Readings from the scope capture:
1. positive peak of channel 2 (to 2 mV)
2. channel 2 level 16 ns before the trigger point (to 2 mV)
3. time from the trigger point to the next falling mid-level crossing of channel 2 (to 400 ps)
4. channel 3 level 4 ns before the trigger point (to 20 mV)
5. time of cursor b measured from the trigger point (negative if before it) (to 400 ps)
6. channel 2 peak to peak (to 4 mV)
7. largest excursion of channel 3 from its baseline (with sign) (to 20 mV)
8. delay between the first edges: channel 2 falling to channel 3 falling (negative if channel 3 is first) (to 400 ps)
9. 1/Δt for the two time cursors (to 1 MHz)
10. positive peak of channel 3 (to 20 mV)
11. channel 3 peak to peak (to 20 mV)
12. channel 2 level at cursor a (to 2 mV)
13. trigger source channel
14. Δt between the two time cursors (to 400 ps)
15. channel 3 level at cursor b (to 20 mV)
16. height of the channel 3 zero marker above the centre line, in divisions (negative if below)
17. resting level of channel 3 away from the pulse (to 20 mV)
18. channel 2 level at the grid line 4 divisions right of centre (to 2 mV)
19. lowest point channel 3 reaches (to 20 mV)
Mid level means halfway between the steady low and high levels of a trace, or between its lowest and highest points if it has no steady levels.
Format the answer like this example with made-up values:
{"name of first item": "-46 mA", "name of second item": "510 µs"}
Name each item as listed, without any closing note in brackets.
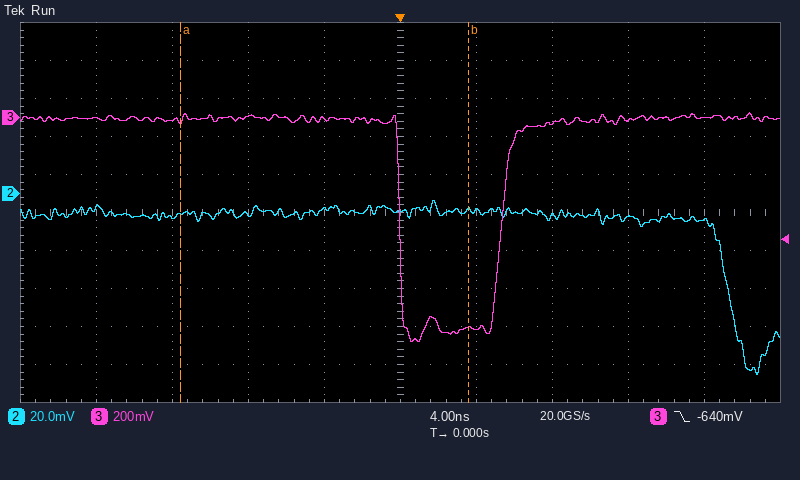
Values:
{"positive peak of channel 2": "-4 mV", "channel 2 level 16 ns before the trigger point": "-8 mV", "time from the trigger point to the next falling mid-level crossing of channel 2": "17.2 ns", "channel 3 level 4 ns before the trigger point": "0 mV", "time of cursor b measured from the trigger point (negative if before it)": "+3.6 ns", "channel 2 peak to peak": "92 mV", "largest excursion of channel 3 from its baseline (with sign)": "-1.18 V", "delay between the first edges: channel 2 falling to channel 3 falling (negative if channel 3 is first)": "-17.2 ns", "1/Δt for the two time cursors": "66 MHz", "positive peak of channel 3": "20 mV", "channel 3 peak to peak": "1.20 V", "channel 2 level at cursor a": "-10 mV", "trigger source channel": "channel 3", "Δt between the two time cursors": "15.2 ns", "channel 3 level at cursor b": "-1.10 V", "height of the channel 3 zero marker above the centre line, in divisions": "+2.5 div", "resting level of channel 3 away from the pulse": "0 mV", "channel 2 level at the grid line 4 divisions right of centre": "-14 mV", "lowest point channel 3 reaches": "-1.18 V"}
